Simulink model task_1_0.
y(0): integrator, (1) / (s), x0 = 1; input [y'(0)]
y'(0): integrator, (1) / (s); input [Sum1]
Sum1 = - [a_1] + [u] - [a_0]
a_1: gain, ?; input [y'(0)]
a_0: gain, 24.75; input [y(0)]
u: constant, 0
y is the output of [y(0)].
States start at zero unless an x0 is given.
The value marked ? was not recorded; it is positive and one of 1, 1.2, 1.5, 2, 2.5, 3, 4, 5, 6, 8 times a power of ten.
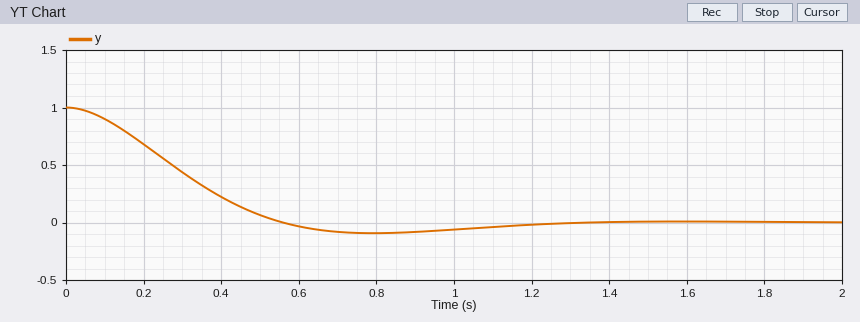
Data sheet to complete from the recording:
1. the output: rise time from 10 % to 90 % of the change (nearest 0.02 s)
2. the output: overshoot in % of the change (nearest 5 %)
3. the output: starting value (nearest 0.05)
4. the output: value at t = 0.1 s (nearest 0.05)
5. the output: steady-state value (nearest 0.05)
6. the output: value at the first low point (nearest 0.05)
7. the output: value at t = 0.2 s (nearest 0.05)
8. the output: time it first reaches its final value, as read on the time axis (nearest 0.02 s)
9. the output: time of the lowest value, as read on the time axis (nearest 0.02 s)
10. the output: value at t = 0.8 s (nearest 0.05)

0.38 s
10 %
1.00
0.90
0.00
-0.10
0.70
0.56 s
0.80 s
-0.10
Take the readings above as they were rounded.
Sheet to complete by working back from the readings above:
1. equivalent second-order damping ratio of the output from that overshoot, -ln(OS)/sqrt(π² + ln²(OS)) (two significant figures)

0.59
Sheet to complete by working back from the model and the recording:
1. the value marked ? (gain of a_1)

6
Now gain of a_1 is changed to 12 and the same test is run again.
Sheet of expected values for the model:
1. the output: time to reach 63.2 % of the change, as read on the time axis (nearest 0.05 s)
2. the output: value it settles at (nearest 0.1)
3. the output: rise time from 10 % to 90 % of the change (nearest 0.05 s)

0.50 s
0.0
0.90 s
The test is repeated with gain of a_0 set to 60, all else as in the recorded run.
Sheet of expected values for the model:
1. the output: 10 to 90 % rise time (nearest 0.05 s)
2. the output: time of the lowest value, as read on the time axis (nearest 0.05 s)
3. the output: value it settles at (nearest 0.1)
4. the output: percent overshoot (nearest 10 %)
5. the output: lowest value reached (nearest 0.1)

0.20 s
0.45 s
0.0
30 %
-0.3
